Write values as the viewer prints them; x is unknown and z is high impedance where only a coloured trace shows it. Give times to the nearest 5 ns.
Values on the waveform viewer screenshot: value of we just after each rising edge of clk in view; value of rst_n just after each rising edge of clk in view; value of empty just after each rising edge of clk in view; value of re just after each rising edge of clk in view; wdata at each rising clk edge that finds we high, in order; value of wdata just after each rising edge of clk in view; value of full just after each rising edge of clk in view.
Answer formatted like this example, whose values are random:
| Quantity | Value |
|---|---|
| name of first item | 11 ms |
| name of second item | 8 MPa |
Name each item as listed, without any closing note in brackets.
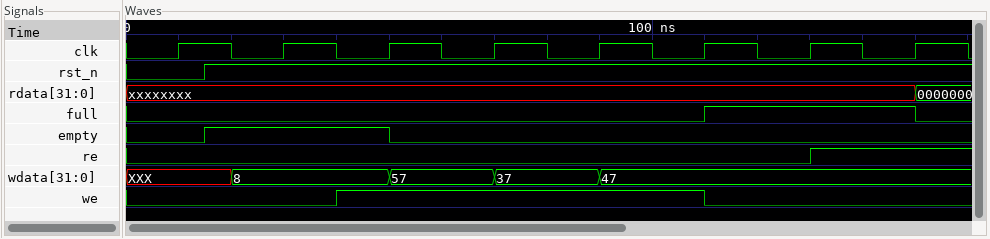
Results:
| Quantity | Value |
|---|---|
| value of we just after each rising edge of clk in view | 0 0 1 1 1 0 0 0 |
| value of rst_n just after each rising edge of clk in view | 0 1 1 1 1 1 1 1 |
| value of empty just after each rising edge of clk in view | 0 1 0 0 0 0 0 0 |
| value of re just after each rising edge of clk in view | 0 0 0 0 0 0 1 1 |
| wdata at each rising clk edge that finds we high, in order | 8, 57, 37, 47 |
| value of wdata just after each rising edge of clk in view | XXX, 8, 57, 37, 47, 47, 47, 47 |
| value of full just after each rising edge of clk in view | 0 0 0 0 0 1 1 0 |
